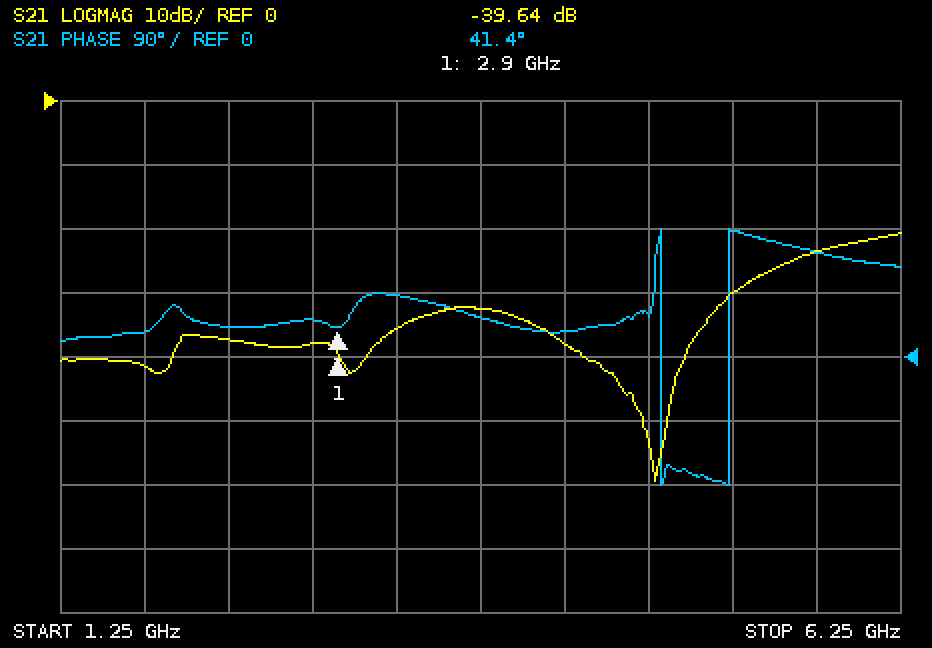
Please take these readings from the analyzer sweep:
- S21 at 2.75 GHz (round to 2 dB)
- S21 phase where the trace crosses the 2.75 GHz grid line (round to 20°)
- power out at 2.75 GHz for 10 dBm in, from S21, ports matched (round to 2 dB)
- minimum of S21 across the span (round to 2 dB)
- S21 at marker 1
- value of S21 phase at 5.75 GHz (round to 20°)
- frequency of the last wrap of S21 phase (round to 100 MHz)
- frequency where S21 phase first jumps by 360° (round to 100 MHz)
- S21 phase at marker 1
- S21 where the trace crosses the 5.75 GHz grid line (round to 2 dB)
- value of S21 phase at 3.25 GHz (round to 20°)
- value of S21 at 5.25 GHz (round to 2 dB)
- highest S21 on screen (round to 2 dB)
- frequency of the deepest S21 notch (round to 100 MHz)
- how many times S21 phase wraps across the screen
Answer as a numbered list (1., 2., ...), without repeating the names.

1. -38 dB
2. 60°
3. -28 dBm
4. -60 dB
5. -39.64 dB
6. 140°
7. 5.2 GHz
8. 4.8 GHz
9. 41.4°
10. -24 dB
11. 80°
12. -30 dB
13. -20 dB
14. 4.8 GHz
15. 2
